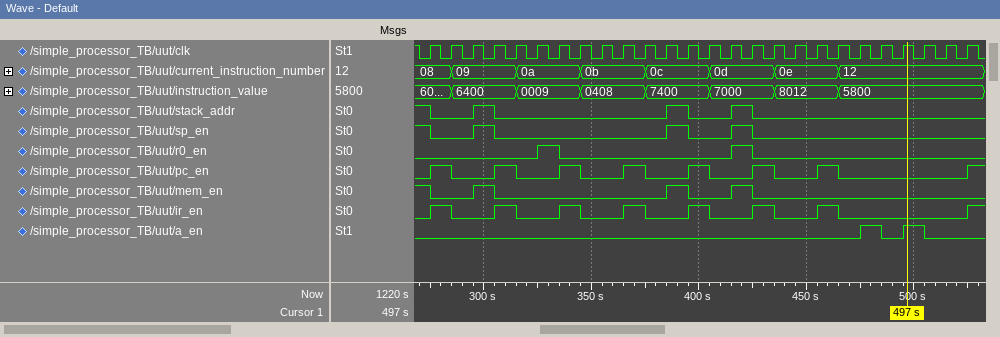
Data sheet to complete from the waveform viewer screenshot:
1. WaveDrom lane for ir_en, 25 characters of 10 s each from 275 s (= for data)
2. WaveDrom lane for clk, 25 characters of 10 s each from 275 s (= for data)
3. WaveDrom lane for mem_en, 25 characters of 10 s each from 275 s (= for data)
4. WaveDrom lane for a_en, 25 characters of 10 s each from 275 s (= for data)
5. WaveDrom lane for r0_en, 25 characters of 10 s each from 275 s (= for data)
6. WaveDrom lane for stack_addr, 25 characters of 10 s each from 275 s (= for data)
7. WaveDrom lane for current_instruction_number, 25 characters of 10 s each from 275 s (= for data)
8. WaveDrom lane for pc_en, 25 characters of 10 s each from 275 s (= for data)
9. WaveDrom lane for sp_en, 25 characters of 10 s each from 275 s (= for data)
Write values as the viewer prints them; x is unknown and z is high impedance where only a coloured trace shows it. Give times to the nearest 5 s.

{name: 'ir_en', wave: '10.10.10.10.10.10.10.....'}
{name: 'clk', wave: 'p........................'}
{name: 'mem_en', wave: '0.10.......10.10.........'}
{name: 'a_en', wave: '0...................1010.'}
{name: 'r0_en', wave: '0....10.......10.........'}
{name: 'stack_addr', wave: '0.10.......10.10.........'}
{name: 'current_instruction_number', wave: '==..=..=..=..=..=..=.....', data: '08 09 0a 0b 0c 0d 0e 12'}
{name: 'pc_en', wave: '10.10.10.10.10.10.10.....'}
{name: 'sp_en', wave: '0.10.......10.10.........'}
